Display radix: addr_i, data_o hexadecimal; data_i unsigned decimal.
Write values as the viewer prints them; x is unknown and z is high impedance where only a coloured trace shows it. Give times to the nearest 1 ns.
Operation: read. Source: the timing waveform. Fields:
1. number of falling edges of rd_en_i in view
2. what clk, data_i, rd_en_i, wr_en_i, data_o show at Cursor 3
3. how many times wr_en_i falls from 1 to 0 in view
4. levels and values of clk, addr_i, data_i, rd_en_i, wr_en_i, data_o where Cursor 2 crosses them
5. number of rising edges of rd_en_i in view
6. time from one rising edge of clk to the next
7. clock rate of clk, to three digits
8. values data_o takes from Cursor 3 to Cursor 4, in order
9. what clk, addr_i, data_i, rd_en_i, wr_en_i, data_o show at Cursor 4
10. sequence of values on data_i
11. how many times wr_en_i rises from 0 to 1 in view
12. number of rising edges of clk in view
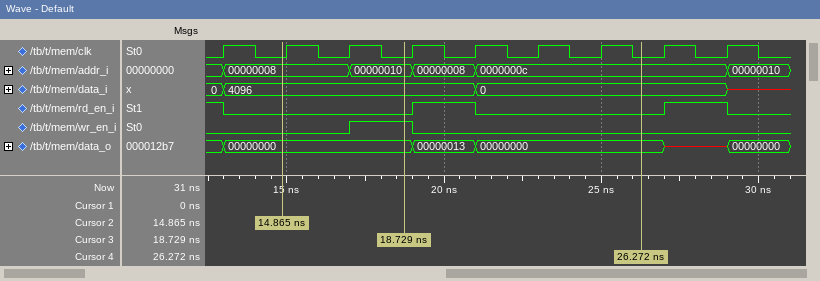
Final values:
3
clk=0, data_i=4096, rd_en_i=0, wr_en_i=1, data_o=00000000
1
clk=0, addr_i=00000008, data_i=4096, rd_en_i=0, wr_en_i=0, data_o=00000000
2
2 ns
500 MHz
00000000, 00000013, 00000000
clk=0, addr_i=0000000c, data_i=0, rd_en_i=0, wr_en_i=0, data_o=00000000
0, 4096, 0, x
1
9
